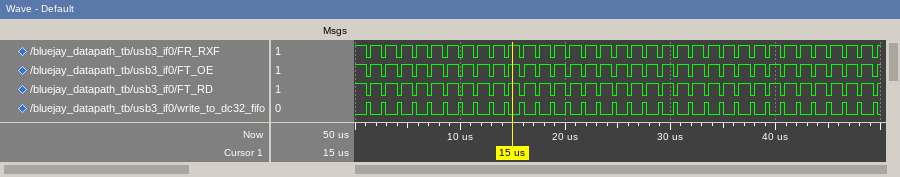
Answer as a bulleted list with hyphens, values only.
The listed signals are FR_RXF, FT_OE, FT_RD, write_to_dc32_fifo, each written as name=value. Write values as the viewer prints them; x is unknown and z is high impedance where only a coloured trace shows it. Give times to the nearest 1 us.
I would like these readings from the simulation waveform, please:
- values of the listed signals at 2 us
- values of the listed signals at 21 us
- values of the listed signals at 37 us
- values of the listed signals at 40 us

- FR_RXF=1, FT_OE=1, FT_RD=1, write_to_dc32_fifo=0
- FR_RXF=1, FT_OE=1, FT_RD=1, write_to_dc32_fifo=0
- FR_RXF=1, FT_OE=1, FT_RD=1, write_to_dc32_fifo=0
- FR_RXF=1, FT_OE=1, FT_RD=1, write_to_dc32_fifo=0
